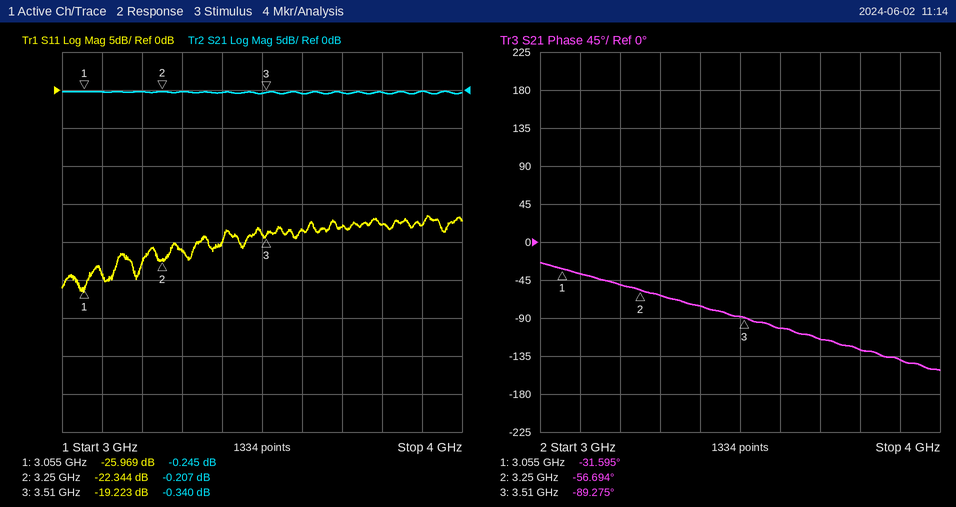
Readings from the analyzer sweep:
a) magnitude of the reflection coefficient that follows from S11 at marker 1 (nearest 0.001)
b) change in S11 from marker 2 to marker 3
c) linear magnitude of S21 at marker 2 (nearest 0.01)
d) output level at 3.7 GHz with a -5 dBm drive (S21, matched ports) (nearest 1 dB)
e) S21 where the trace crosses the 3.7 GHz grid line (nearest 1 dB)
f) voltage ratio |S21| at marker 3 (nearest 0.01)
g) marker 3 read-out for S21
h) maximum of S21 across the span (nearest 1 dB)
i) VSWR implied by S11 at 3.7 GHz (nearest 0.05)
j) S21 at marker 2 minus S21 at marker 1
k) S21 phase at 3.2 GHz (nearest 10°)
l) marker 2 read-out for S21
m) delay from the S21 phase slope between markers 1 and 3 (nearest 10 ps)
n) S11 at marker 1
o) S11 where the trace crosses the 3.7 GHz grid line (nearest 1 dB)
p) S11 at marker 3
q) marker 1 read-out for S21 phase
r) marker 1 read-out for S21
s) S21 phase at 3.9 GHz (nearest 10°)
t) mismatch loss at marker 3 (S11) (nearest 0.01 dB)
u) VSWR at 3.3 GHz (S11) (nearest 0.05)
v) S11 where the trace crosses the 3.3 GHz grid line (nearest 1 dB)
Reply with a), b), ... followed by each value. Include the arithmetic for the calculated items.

a) 10^(-25.969/20) ≈ 0.050
b) -19.223 − (-22.344) = 3.121 dB
c) 10^(-0.207/20) ≈ 0.98
d) -5 dBm + (0 dB) = -5 dBm
e) 0 dB
f) 10^(-0.34/20) ≈ 0.96
g) -0.340 dB
h) 0 dB
i) |Γ| = 10^(-18/20) = 0.1259; VSWR = (1 + 0.1259)/(1 − 0.1259) ≈ 1.29, so 1.30 to the nearest 0.05
j) -0.207 − (-0.245) = 0.038 dB
k) -50°
l) -0.207 dB
m) −(-89.275° − (-31.595°))/(360° × 455 MHz) ≈ 352 ps, so 350 ps to the nearest 10 ps
n) -25.969 dB
o) -18 dB
p) -19.223 dB
q) -31.595°
r) -0.245 dB
s) -140°
t) −10 log10(1 − 10^(-19.223/10)) ≈ 0.05 dB
u) |Γ| = 10^(-21/20) = 0.0891; VSWR = (1 + 0.0891)/(1 − 0.0891) ≈ 1.20
v) -21 dB
